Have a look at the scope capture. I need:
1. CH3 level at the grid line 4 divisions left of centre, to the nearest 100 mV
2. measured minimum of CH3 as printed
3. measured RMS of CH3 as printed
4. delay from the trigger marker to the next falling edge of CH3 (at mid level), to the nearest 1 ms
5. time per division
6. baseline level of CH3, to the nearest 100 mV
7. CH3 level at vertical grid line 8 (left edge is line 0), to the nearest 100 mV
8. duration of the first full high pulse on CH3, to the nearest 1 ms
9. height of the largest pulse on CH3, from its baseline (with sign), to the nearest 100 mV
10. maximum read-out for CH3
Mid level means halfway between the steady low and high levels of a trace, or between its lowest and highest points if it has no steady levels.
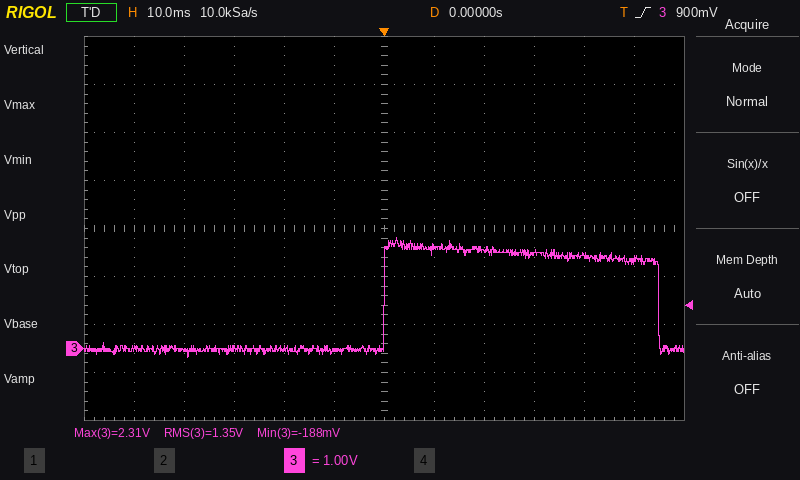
0.0 V
-188 mV
1.35 V
55 ms
10 ms
0.0 V
2.1 V
55 ms
+2.3 V
2.31 V
